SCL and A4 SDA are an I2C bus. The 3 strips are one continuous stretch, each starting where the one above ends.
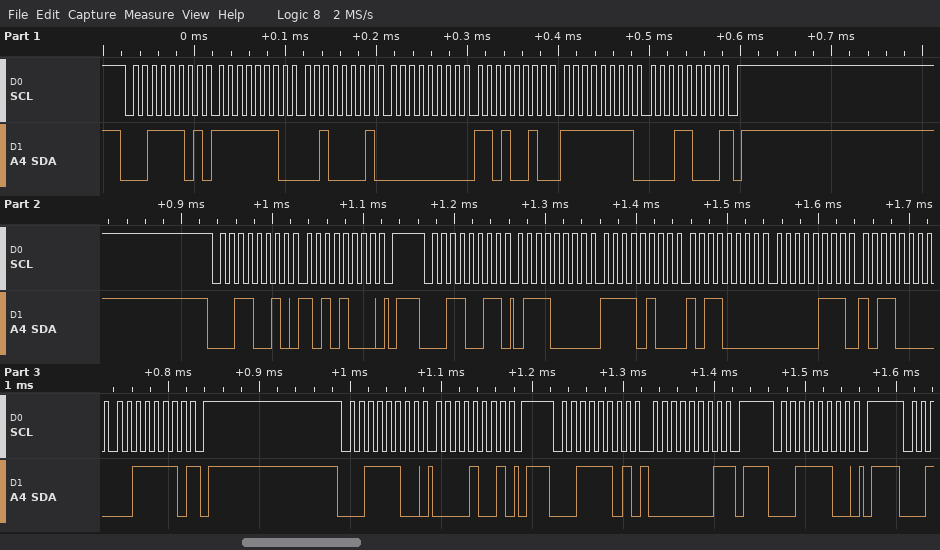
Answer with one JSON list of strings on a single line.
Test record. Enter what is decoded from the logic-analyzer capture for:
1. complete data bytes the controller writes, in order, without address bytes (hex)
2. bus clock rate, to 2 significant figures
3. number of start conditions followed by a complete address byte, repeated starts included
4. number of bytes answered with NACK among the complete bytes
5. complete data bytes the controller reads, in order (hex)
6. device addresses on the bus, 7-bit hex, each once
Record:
["A8 09", "100 kHz", "6", "3", "FE 21 00 D2 FF 18 70 F4 B0 07 B0 3E 01", "0x1E 0x19"]
